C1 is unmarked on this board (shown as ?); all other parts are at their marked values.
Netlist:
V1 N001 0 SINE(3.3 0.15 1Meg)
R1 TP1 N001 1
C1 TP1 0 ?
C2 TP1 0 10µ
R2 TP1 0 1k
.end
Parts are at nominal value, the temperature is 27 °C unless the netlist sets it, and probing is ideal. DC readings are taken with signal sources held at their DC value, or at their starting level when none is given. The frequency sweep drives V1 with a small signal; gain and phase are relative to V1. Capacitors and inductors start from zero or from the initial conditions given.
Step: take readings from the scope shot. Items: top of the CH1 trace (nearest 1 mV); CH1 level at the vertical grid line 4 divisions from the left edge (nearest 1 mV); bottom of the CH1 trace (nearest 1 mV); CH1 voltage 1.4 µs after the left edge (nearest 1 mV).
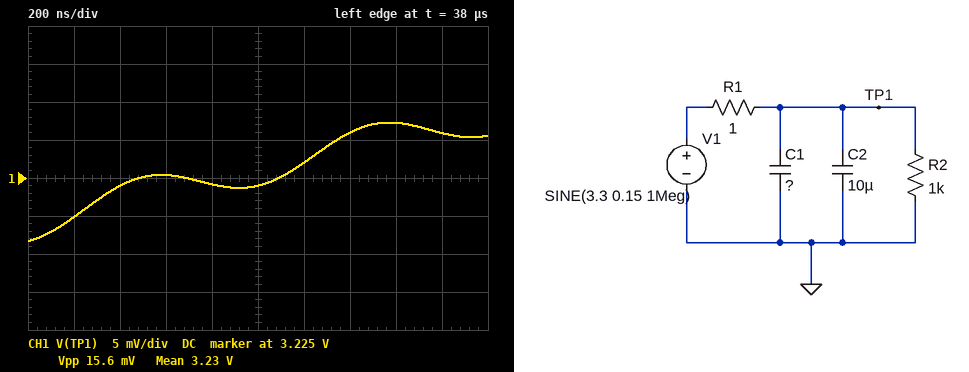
3.232 V
3.224 V
3.217 V
3.231 V
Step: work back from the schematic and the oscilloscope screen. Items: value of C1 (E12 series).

150 nF
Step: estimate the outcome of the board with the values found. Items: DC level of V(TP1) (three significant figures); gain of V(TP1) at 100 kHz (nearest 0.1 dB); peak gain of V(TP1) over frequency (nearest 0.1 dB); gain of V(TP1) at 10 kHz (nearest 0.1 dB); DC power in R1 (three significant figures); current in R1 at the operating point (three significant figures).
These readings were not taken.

3.30 V
-16.2 dB
0 dB
-1.5 dB
10.9 µW
3.30 mA
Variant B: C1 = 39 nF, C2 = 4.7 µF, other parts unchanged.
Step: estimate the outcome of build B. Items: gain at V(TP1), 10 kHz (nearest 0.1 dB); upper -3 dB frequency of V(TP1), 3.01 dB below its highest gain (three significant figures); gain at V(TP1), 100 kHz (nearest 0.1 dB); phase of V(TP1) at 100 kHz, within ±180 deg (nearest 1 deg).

-0.4 dB
33.6 kHz
-9.9 dB
-71 deg
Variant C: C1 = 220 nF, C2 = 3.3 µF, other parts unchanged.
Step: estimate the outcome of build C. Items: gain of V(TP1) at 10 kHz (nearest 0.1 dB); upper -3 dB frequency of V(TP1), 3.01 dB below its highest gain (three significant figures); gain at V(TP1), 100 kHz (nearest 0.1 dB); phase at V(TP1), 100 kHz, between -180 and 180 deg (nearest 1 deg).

-0.2 dB
45.3 kHz
-7.7 dB
-66 deg
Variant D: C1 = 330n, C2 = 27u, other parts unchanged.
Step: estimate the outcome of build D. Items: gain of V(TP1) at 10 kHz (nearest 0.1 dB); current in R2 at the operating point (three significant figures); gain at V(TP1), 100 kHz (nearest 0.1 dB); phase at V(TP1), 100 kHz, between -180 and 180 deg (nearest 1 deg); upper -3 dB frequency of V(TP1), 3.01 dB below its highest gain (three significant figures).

-6.0 dB
3.30 mA
-24.7 dB
-87 deg
5.83 kHz
